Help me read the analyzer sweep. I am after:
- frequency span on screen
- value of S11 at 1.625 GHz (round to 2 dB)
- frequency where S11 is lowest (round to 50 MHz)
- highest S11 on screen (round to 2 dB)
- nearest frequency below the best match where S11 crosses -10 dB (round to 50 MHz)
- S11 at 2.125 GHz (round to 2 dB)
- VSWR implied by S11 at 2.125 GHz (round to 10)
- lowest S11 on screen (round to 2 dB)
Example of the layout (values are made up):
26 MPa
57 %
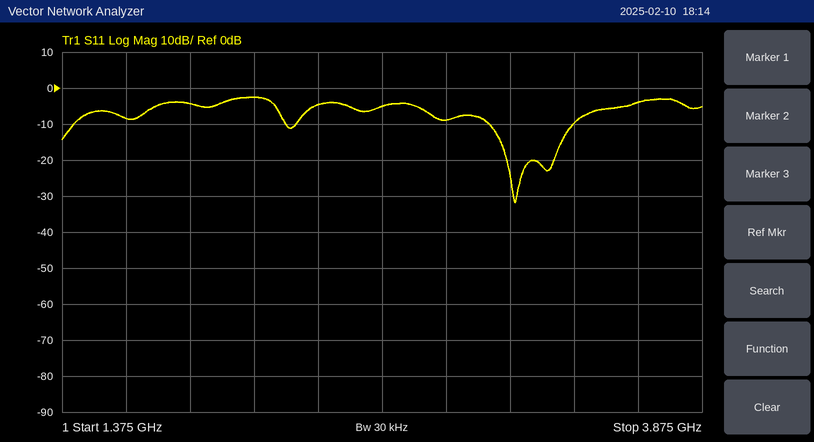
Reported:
2.5 GHz
-8 dB
3.15 GHz
-2 dB
3.05 GHz
-2 dB
10
-32 dB
